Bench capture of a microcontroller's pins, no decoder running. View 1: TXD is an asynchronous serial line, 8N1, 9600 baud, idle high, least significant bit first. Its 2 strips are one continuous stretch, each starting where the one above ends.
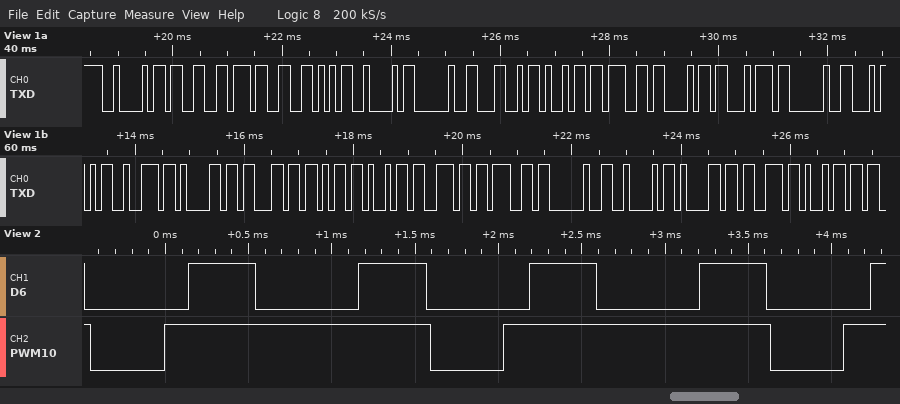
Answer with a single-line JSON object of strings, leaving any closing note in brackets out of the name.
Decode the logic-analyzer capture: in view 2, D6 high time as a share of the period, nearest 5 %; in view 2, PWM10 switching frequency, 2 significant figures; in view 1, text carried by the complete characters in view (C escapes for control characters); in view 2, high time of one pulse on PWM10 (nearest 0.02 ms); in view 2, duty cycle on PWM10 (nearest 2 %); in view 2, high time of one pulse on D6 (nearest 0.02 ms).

{"in view 2, D6 high time as a share of the period, nearest 5 %": "40 %", "in view 2, PWM10 switching frequency, 2 significant figures": "490 Hz", "in view 1, text carried by the complete characters in view": "\"B37VB Light Tracking Basi\"", "in view 2, high time of one pulse on PWM10": "1.60 ms", "in view 2, duty cycle on PWM10": "78 %", "in view 2, high time of one pulse on D6": "0.40 ms"}
